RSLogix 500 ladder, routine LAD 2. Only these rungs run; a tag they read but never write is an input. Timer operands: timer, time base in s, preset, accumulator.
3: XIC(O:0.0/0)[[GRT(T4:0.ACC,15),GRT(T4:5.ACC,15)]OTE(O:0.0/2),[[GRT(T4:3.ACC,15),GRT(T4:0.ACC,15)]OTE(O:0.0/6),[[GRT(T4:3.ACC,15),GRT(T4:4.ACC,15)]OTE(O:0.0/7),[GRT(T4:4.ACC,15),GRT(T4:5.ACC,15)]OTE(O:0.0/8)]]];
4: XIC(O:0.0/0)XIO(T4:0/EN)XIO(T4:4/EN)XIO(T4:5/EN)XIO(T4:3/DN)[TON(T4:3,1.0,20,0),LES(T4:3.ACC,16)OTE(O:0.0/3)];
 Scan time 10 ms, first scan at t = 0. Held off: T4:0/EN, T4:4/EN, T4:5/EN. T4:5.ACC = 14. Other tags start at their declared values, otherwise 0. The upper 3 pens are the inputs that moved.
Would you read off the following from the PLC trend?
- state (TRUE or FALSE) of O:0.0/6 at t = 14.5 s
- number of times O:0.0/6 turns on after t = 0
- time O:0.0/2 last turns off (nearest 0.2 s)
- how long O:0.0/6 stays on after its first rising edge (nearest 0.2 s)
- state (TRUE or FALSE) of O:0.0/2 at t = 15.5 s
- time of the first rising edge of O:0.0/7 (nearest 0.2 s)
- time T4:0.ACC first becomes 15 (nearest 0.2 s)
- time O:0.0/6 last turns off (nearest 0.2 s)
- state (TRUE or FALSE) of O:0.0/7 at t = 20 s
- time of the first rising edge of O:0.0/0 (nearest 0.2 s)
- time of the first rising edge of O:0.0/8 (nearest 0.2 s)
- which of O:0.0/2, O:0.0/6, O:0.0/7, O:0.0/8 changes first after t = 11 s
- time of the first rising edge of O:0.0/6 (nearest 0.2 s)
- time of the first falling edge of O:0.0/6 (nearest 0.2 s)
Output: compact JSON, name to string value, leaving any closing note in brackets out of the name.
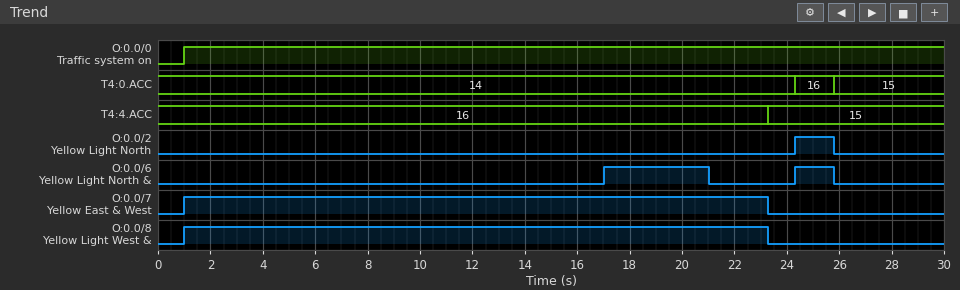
{"state (TRUE or FALSE) of O:0.0/6 at t = 14.5 s": "FALSE", "number of times O:0.0/6 turns on after t = 0": "2", "time O:0.0/2 last turns off": "25.8 s", "how long O:0.0/6 stays on after its first rising edge": "4.0 s", "state (TRUE or FALSE) of O:0.0/2 at t = 15.5 s": "FALSE", "time of the first rising edge of O:0.0/7": "1.0 s", "time T4:0.ACC first becomes 15": "25.8 s", "time O:0.0/6 last turns off": "25.8 s", "state (TRUE or FALSE) of O:0.0/7 at t = 20 s": "TRUE", "time of the first rising edge of O:0.0/0": "1.0 s", "time of the first rising edge of O:0.0/8": "1.0 s", "which of O:0.0/2, O:0.0/6, O:0.0/7, O:0.0/8 changes first after t = 11 s": "O:0.0/6", "time of the first rising edge of O:0.0/6": "17.0 s", "time of the first falling edge of O:0.0/6": "21.0 s"}
